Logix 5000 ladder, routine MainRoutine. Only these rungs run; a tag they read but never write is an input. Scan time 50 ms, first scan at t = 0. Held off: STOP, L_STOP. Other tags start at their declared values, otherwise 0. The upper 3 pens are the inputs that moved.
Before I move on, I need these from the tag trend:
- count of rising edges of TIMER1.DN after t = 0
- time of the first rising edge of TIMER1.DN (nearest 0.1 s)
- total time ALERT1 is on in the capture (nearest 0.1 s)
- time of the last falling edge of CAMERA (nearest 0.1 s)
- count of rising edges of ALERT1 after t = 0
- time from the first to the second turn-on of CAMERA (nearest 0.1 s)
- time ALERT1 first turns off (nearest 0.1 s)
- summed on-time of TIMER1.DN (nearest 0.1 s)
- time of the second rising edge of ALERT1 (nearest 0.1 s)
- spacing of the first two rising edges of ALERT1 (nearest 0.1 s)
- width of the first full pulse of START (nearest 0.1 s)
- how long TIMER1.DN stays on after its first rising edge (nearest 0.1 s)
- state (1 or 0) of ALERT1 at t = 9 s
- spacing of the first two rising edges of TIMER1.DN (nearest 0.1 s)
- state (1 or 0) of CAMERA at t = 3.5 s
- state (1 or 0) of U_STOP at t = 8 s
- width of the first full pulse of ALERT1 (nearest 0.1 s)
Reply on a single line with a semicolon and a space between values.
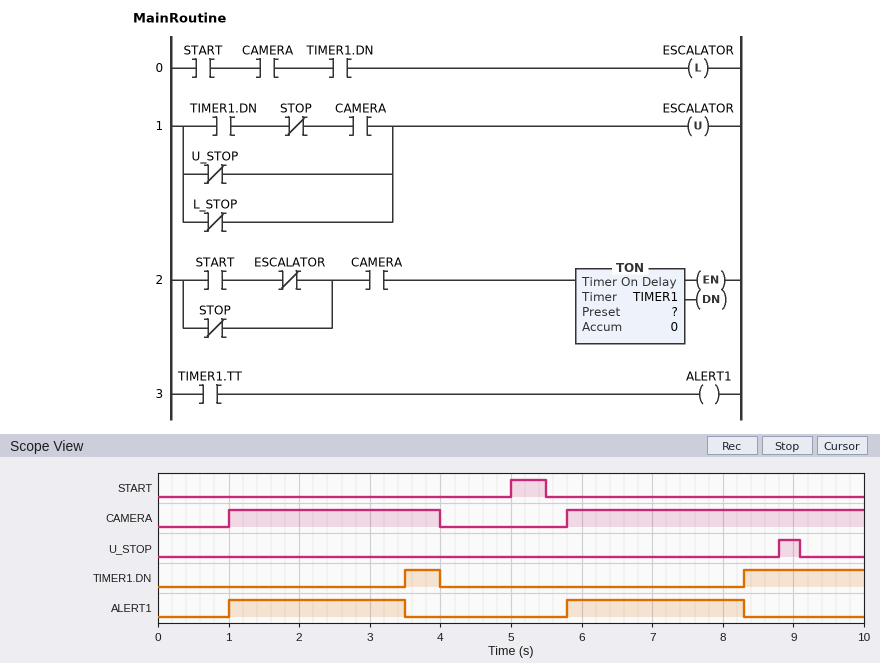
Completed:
2; 3.5 s; 5.0 s; 4.0 s; 2; 4.8 s; 3.5 s; 2.2 s; 5.8 s; 4.8 s; 0.5 s; 0.5 s; 0; 4.8 s; 1; 0; 2.5 s
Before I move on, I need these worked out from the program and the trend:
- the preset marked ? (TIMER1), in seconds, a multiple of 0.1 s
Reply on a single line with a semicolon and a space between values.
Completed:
2.5 s
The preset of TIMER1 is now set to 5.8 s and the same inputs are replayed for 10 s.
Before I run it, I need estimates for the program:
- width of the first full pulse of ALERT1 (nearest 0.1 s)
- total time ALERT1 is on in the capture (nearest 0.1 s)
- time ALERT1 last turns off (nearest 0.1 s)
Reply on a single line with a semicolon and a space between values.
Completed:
3.0 s; 7.2 s; 4.0 s
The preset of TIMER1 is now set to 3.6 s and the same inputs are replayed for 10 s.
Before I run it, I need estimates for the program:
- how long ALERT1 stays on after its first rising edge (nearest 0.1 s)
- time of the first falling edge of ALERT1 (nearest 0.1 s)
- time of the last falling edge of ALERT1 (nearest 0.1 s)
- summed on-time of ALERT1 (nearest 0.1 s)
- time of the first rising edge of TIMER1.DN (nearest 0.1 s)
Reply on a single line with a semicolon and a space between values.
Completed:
3.0 s; 4.0 s; 9.4 s; 6.6 s; 9.4 s
